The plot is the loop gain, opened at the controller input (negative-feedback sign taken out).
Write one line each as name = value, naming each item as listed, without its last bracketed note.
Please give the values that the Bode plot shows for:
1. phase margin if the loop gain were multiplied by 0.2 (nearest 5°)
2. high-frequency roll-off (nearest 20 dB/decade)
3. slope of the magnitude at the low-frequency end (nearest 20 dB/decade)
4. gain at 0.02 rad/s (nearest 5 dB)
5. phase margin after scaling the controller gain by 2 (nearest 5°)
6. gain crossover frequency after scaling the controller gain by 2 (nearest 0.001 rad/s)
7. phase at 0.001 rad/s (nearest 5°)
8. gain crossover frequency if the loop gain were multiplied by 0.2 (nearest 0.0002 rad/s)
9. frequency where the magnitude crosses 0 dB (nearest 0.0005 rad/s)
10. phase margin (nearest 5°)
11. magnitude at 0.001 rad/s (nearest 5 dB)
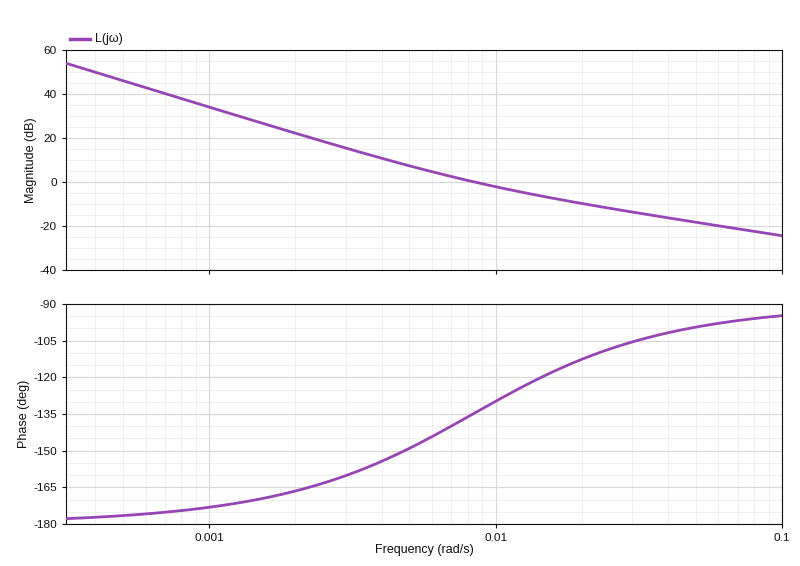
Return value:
phase margin if the loop gain were multiplied by 0.2 = 20°
high-frequency roll-off = -20 dB/decade
slope of the magnitude at the low-frequency end = -40 dB/decade
gain at 0.02 rad/s = -10 dB
phase margin after scaling the controller gain by 2 = 60°
gain crossover frequency after scaling the controller gain by 2 = 0.014 rad/s
phase at 0.001 rad/s = -175°
gain crossover frequency if the loop gain were multiplied by 0.2 = 0.0032 rad/s
frequency where the magnitude crosses 0 dB = 0.0085 rad/s
phase margin = 45°
magnitude at 0.001 rad/s = 35 dB
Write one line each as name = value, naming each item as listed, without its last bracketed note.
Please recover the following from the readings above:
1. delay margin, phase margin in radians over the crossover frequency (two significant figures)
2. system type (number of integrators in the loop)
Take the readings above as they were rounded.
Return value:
delay margin, phase margin in radians over the crossover frequency = 92 s
system type = 2
